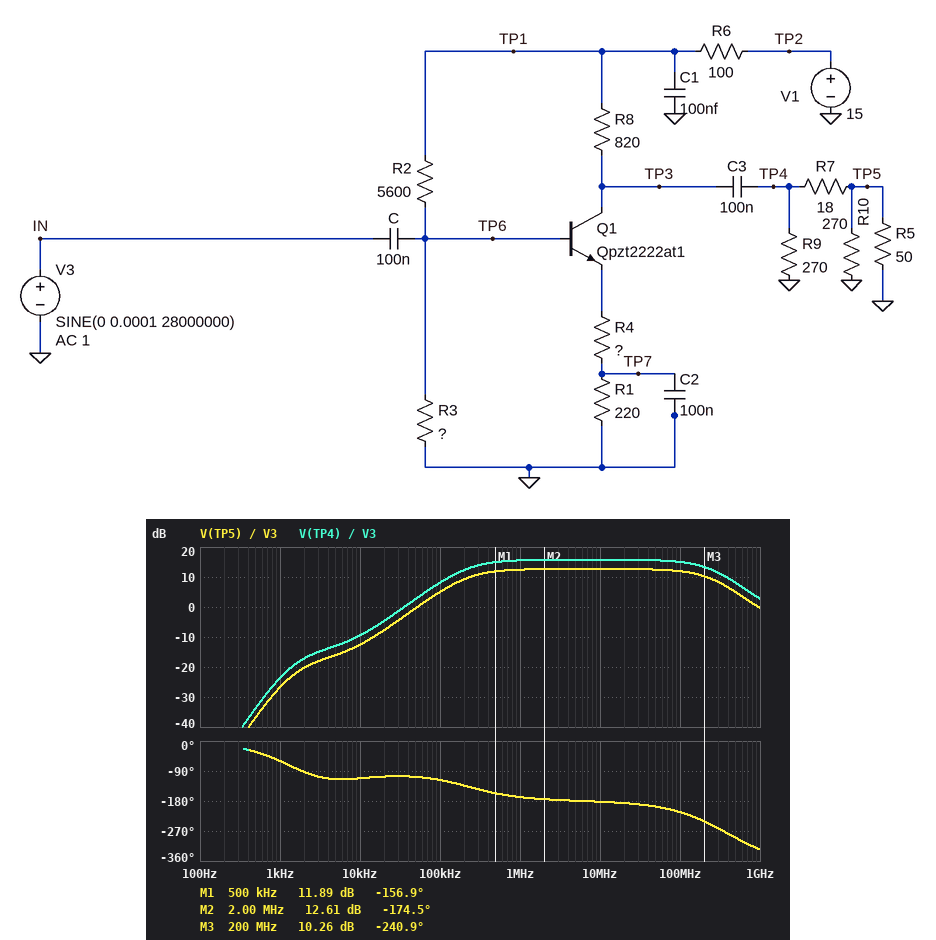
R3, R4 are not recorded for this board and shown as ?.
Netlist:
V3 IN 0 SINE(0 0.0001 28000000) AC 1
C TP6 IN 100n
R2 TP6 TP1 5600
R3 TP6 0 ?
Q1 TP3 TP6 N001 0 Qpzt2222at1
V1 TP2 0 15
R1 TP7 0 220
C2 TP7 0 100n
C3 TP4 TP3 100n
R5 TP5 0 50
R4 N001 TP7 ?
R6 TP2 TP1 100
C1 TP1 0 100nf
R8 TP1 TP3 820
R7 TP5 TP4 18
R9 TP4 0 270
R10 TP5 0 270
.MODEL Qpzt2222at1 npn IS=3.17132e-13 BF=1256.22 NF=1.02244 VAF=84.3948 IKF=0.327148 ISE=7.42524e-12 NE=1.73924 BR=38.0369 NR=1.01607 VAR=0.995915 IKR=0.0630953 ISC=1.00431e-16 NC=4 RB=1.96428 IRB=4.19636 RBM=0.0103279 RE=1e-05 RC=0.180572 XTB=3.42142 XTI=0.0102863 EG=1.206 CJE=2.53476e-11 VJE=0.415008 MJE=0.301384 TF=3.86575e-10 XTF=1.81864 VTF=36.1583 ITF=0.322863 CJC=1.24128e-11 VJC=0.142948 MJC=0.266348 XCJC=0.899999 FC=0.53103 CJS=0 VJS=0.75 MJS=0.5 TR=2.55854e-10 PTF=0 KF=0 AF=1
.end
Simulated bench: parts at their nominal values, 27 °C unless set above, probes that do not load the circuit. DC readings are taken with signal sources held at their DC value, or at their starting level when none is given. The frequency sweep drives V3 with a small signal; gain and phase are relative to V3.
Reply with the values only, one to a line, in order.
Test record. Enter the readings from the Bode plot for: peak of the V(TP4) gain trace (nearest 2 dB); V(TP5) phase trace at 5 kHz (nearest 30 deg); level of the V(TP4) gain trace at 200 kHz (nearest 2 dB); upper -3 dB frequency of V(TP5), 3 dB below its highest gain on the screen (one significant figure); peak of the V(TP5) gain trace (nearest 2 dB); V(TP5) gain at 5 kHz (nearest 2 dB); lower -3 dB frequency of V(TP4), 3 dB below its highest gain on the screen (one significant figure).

16 dB
-120 deg
12 dB
200 MHz
12 dB
-16 dB
200 kHz
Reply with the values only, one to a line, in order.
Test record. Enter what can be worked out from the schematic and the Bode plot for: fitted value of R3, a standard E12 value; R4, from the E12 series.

1.8 kΩ
4.7 Ω
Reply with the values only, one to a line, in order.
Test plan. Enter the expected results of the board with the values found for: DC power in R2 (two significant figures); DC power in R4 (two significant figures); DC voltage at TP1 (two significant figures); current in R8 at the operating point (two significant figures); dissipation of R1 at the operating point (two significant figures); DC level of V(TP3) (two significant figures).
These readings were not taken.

19 mW
620 µW
14 V
11 mA
29 mW
4.3 V
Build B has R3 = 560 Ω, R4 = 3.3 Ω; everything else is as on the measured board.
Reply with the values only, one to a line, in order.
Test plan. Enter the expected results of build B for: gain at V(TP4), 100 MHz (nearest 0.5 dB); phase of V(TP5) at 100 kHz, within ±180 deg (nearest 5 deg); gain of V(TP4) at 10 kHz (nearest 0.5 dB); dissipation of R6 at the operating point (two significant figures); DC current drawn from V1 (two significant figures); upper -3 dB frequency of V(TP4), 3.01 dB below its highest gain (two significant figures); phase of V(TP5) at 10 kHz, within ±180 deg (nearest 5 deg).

11.0 dB
-130 deg
-10.0 dB
2.9 mW
5.4 mA
390 MHz
-105 deg
